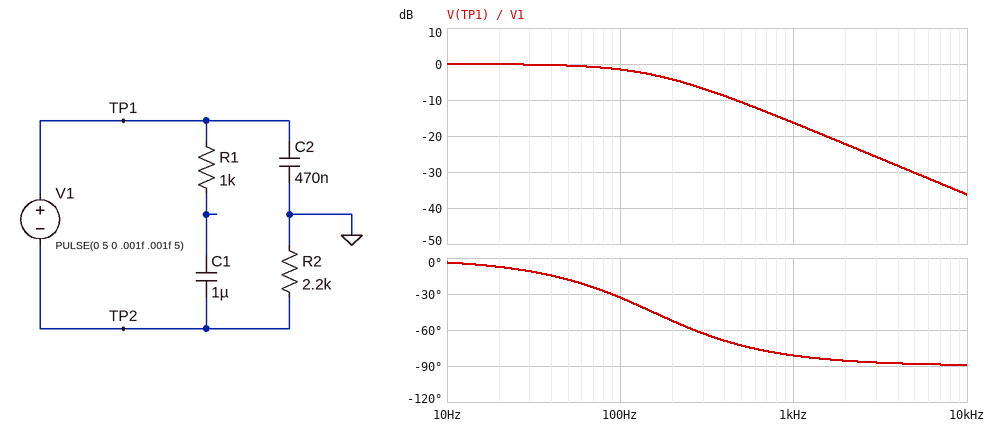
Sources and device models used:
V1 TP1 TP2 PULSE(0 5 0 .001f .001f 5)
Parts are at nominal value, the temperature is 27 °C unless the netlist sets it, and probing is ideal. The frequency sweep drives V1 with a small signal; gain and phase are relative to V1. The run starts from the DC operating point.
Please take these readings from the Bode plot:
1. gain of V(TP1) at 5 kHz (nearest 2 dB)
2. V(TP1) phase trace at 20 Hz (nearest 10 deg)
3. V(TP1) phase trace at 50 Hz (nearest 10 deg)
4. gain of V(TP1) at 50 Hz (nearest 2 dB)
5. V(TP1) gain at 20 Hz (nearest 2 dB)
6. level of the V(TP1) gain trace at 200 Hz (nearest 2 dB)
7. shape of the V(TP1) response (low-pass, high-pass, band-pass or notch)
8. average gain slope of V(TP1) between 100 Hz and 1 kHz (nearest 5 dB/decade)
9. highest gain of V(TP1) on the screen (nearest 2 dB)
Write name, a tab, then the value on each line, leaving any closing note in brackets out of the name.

gain of V(TP1) at 5 kHz	-30 dB
V(TP1) phase trace at 20 Hz	-10 deg
V(TP1) phase trace at 50 Hz	-20 deg
gain of V(TP1) at 50 Hz	0 dB
V(TP1) gain at 20 Hz	0 dB
level of the V(TP1) gain trace at 200 Hz	-4 dB
shape of the V(TP1) response	low-pass
average gain slope of V(TP1) between 100 Hz and 1 kHz	-15 dB/decade
highest gain of V(TP1) on the screen	0 dB
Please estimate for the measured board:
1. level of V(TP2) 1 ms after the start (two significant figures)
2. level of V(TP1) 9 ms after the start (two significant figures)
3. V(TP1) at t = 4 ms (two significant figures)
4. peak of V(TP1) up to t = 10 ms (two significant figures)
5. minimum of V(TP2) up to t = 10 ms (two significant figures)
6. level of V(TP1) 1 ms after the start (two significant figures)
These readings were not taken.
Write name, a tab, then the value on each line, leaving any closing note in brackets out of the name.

level of V(TP2) 1 ms after the start	-1.9 V
level of V(TP1) 9 ms after the start	5.0 V
V(TP1) at t = 4 ms	4.9 V
peak of V(TP1) up to t = 10 ms	5.0 V
minimum of V(TP2) up to t = 10 ms	-5.0 V
level of V(TP1) 1 ms after the start	3.1 V
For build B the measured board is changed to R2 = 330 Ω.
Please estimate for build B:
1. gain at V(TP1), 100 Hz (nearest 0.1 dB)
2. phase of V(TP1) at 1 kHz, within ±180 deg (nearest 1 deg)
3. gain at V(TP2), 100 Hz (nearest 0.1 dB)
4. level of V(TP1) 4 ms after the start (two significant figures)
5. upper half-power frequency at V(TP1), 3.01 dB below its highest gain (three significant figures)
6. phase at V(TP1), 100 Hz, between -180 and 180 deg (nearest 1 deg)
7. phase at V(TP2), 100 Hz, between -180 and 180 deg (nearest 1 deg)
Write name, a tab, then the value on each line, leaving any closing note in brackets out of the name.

gain at V(TP1), 100 Hz	0 dB
phase of V(TP1) at 1 kHz, within ±180 deg	-44 deg
gain at V(TP2), 100 Hz	-20.3 dB
level of V(TP1) 4 ms after the start	5.0 V
upper half-power frequency at V(TP1), 3.01 dB below its highest gain	1.03 kHz
phase at V(TP1), 100 Hz, between -180 and 180 deg	-6 deg
phase at V(TP2), 100 Hz, between -180 and 180 deg	-96 deg
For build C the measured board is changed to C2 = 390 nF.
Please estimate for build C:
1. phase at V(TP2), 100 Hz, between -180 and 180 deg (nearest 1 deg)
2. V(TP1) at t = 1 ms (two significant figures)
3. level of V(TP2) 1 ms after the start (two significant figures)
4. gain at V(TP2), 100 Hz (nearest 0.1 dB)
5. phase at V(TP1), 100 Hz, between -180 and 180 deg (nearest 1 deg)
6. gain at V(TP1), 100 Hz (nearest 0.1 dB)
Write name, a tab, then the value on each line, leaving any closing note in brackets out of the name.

phase at V(TP2), 100 Hz, between -180 and 180 deg	-118 deg
V(TP1) at t = 1 ms	3.4 V
level of V(TP2) 1 ms after the start	-1.6 V
gain at V(TP2), 100 Hz	-6.5 dB
phase at V(TP1), 100 Hz, between -180 and 180 deg	-28 deg
gain at V(TP1), 100 Hz	-1.1 dB
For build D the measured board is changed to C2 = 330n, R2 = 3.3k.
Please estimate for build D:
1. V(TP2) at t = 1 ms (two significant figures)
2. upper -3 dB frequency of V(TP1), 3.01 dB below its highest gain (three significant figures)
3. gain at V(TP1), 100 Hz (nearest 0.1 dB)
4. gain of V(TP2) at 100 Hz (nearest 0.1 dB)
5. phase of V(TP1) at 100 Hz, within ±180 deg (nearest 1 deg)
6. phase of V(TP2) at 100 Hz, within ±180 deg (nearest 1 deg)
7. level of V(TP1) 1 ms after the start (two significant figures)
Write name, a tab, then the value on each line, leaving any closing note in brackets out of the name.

V(TP2) at t = 1 ms	-2.0 V
upper -3 dB frequency of V(TP1), 3.01 dB below its highest gain	146 Hz
gain at V(TP1), 100 Hz	-1.7 dB
gain of V(TP2) at 100 Hz	-5.0 dB
phase of V(TP1) at 100 Hz, within ±180 deg	-34 deg
phase of V(TP2) at 100 Hz, within ±180 deg	-124 deg
level of V(TP1) 1 ms after the start	3.0 V
